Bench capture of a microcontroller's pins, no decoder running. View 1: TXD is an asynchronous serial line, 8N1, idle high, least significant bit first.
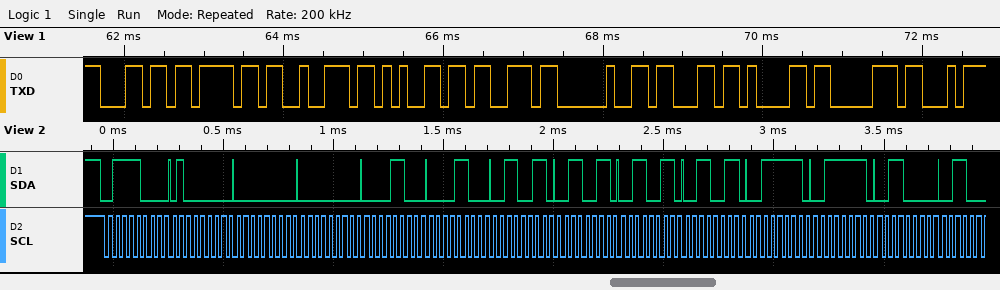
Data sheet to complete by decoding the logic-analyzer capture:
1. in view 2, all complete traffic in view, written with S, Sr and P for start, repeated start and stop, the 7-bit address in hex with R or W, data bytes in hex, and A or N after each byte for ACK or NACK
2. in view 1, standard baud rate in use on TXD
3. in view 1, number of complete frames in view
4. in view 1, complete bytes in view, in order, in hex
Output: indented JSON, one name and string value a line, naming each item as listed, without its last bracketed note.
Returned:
{
  "in view 2, all complete traffic in view, written with S, Sr and P for start, repeated start and stop, the 7-bit address in hex with R or W, data bytes in hex, and A or N after each byte for ACK or NACK": "S 3CW A 40 A 00 A 00 A 0C A 0C A 33 A 33 A 33 A 33 A 3F A 3F A 30 A",
  "in view 1, standard baud rate in use on TXD": "9600 baud",
  "in view 1, number of complete frames in view": "9",
  "in view 1, complete bytes in view, in order, in hex": "6C 6F 72 65 73 20 63 61 70"
}
